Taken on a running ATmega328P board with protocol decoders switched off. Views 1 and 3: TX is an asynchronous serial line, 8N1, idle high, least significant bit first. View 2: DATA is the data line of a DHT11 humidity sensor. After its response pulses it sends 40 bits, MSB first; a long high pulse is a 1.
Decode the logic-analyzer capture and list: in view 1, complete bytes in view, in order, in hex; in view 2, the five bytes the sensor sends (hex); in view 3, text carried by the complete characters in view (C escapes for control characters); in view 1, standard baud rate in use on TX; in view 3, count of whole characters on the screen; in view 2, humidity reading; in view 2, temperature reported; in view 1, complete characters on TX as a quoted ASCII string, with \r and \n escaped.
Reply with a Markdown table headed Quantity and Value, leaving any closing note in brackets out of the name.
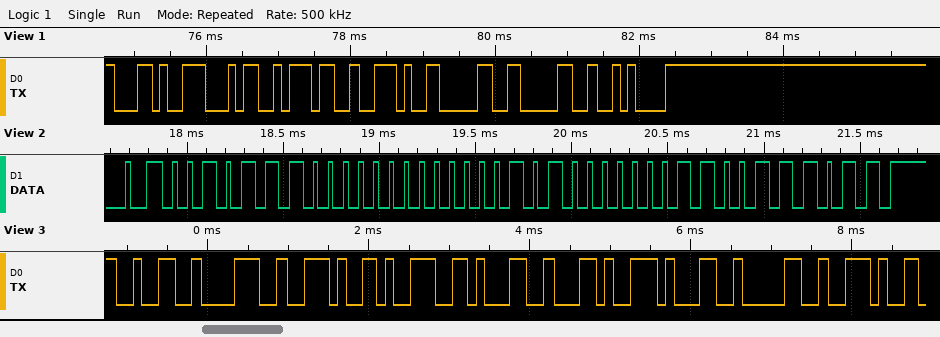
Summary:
| Quantity | Value |
|---|---|
| in view 1, complete bytes in view, in order, in hex | 2C 34 37 2E 30 30 0A |
| in view 2, the five bytes the sensor sends | 2E 00 0A 03 3B |
| in view 3, text carried by the complete characters in view | "28.91,10." |
| in view 1, standard baud rate in use on TX | 9600 baud |
| in view 3, count of whole characters on the screen | 9 |
| in view 2, humidity reading | 46 % |
| in view 2, temperature reported | 10.3 °C |
| in view 1, complete characters on TX as a quoted ASCII string, with \r and \n escaped | ",47.00\n" |
